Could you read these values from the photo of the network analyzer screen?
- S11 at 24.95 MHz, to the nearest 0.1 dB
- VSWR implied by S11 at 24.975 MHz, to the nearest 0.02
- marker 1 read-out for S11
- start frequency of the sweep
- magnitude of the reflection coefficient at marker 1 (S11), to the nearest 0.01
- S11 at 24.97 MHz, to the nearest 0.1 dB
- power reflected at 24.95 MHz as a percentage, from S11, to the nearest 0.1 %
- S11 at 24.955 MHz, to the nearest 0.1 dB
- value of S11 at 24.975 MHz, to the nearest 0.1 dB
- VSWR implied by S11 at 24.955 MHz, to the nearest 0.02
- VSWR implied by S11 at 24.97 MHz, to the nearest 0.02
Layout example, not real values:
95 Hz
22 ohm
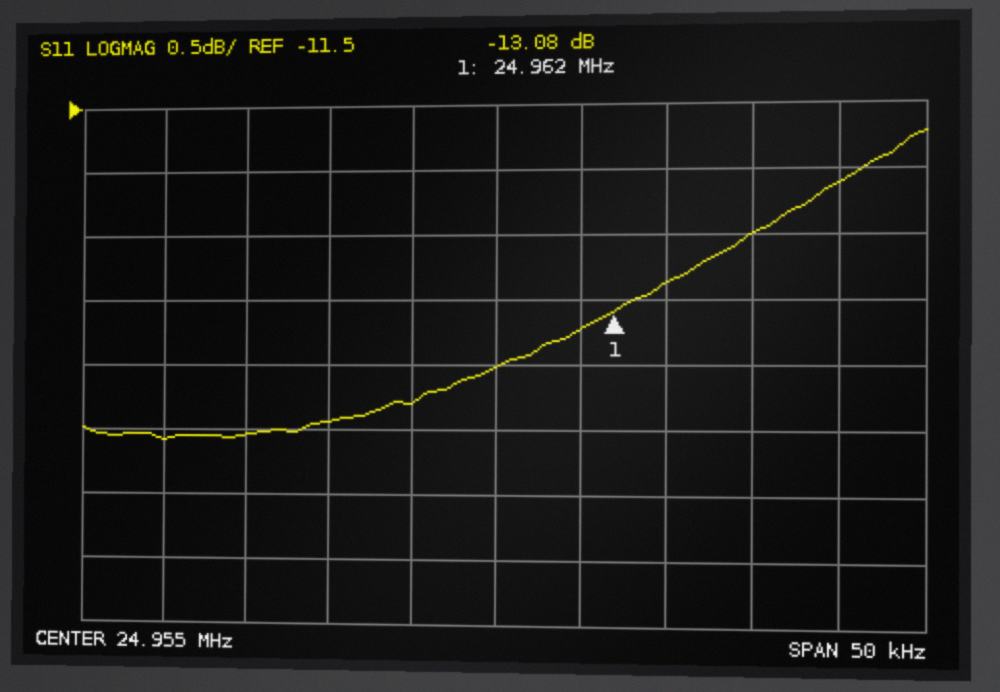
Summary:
-13.8 dB
1.66
-13.08 dB
24.93 MHz
0.22
-12.5 dB
4.2 %
-13.5 dB
-12.1 dB
1.54
1.62
